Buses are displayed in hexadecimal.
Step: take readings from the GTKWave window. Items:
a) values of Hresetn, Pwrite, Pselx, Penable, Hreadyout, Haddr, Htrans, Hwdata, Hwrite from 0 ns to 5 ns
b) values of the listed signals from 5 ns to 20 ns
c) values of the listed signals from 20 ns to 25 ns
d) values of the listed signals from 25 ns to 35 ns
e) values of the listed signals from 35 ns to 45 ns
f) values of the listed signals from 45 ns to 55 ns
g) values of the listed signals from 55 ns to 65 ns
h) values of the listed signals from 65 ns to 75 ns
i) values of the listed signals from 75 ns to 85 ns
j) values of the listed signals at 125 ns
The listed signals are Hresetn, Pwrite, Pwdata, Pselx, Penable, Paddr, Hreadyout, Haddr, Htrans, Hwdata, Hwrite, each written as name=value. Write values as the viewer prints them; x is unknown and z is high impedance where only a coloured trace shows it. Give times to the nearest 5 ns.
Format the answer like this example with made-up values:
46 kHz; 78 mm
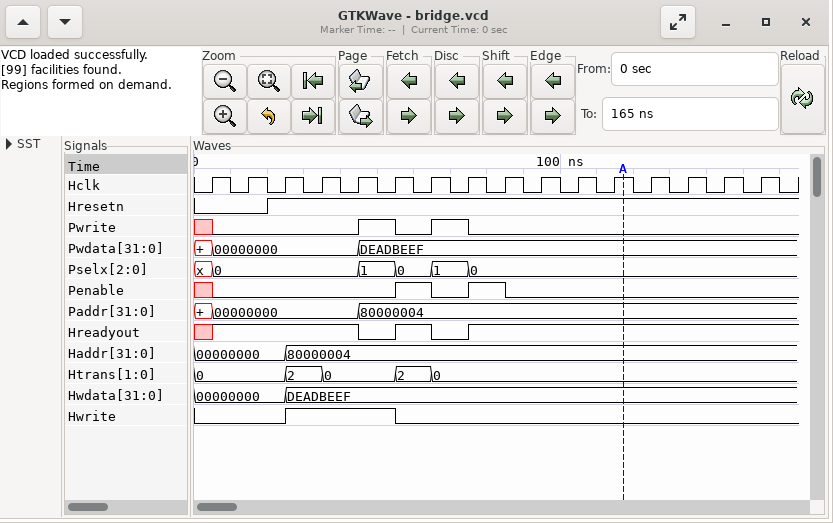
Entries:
Hresetn=0, Pwrite=x, Pselx=x, Penable=x, Hreadyout=x, Haddr=00000000, Htrans=0, Hwdata=00000000, Hwrite=0; Hresetn=0, Pwrite=0, Pwdata=00000000, Pselx=0, Penable=0, Paddr=00000000, Hreadyout=1, Haddr=00000000, Htrans=0, Hwdata=00000000, Hwrite=0; Hresetn=1, Pwrite=0, Pwdata=00000000, Pselx=0, Penable=0, Paddr=00000000, Hreadyout=1, Haddr=00000000, Htrans=0, Hwdata=00000000, Hwrite=0; Hresetn=1, Pwrite=0, Pwdata=00000000, Pselx=0, Penable=0, Paddr=00000000, Hreadyout=1, Haddr=80000004, Htrans=2, Hwdata=DEADBEEF, Hwrite=1; Hresetn=1, Pwrite=0, Pwdata=00000000, Pselx=0, Penable=0, Paddr=00000000, Hreadyout=1, Haddr=80000004, Htrans=0, Hwdata=DEADBEEF, Hwrite=1; Hresetn=1, Pwrite=1, Pwdata=DEADBEEF, Pselx=1, Penable=0, Paddr=80000004, Hreadyout=0, Haddr=80000004, Htrans=0, Hwdata=DEADBEEF, Hwrite=1; Hresetn=1, Pwrite=0, Pwdata=DEADBEEF, Pselx=0, Penable=1, Paddr=80000004, Hreadyout=1, Haddr=80000004, Htrans=2, Hwdata=DEADBEEF, Hwrite=0; Hresetn=1, Pwrite=1, Pwdata=DEADBEEF, Pselx=1, Penable=0, Paddr=80000004, Hreadyout=0, Haddr=80000004, Htrans=0, Hwdata=DEADBEEF, Hwrite=0; Hresetn=1, Pwrite=0, Pwdata=DEADBEEF, Pselx=0, Penable=1, Paddr=80000004, Hreadyout=1, Haddr=80000004, Htrans=0, Hwdata=DEADBEEF, Hwrite=0; Hresetn=1, Pwrite=0, Pwdata=DEADBEEF, Pselx=0, Penable=0, Paddr=80000004, Hreadyout=1, Haddr=80000004, Htrans=0, Hwdata=DEADBEEF, Hwrite=0
